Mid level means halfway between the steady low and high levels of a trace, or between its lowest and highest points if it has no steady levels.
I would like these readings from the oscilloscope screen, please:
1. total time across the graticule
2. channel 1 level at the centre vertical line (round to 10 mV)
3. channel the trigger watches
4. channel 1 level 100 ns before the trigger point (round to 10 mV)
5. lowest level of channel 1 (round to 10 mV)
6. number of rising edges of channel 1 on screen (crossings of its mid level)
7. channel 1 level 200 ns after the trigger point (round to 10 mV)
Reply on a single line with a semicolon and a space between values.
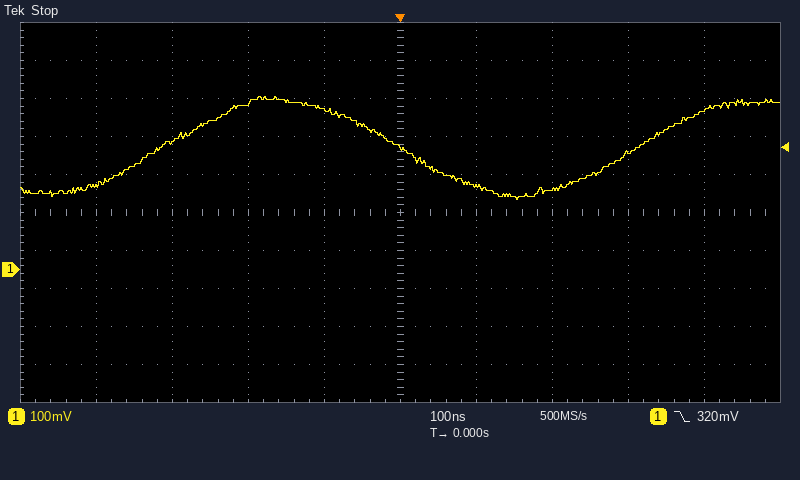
1 µs; 320 mV; channel 1; 420 mV; 180 mV; 2; 210 mV
